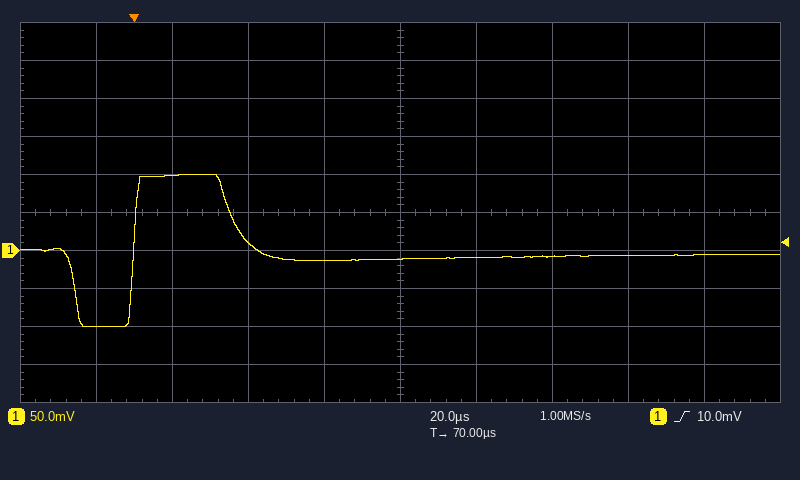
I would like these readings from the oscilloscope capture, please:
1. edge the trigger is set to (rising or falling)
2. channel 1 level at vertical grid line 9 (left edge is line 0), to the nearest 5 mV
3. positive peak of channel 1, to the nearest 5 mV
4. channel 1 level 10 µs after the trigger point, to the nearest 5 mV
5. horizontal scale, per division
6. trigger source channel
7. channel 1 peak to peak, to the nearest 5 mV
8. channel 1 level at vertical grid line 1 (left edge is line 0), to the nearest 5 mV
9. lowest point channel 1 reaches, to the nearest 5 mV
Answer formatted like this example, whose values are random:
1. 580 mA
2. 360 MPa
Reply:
1. rising
2. -5 mV
3. 100 mV
4. 100 mV
5. 20 µs
6. channel 1
7. 200 mV
8. -100 mV
9. -100 mV
